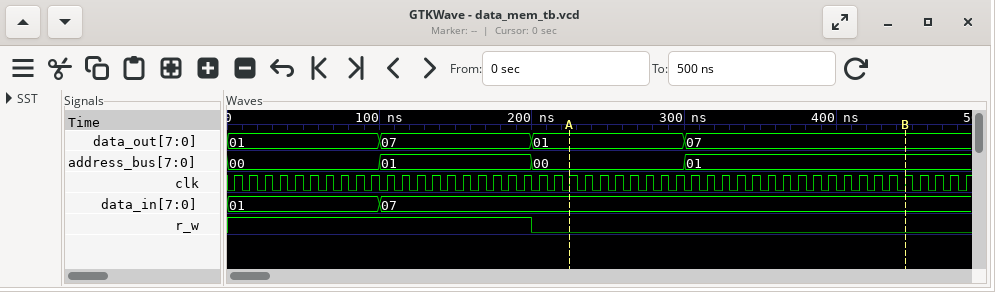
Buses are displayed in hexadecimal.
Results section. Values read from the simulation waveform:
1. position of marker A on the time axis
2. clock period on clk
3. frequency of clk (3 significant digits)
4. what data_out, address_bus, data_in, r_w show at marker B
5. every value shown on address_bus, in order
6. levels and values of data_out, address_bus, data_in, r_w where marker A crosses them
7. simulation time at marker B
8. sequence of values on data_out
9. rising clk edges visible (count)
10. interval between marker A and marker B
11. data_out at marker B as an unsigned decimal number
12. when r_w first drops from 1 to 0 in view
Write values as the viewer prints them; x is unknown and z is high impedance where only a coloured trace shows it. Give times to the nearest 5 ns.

225 ns
10 ns
100 MHz
data_out=07, address_bus=01, data_in=07, r_w=0
00, 01, 00, 01
data_out=01, address_bus=00, data_in=07, r_w=0
445 ns
01, 07, 01, 07
49
220 ns
7
200 ns
